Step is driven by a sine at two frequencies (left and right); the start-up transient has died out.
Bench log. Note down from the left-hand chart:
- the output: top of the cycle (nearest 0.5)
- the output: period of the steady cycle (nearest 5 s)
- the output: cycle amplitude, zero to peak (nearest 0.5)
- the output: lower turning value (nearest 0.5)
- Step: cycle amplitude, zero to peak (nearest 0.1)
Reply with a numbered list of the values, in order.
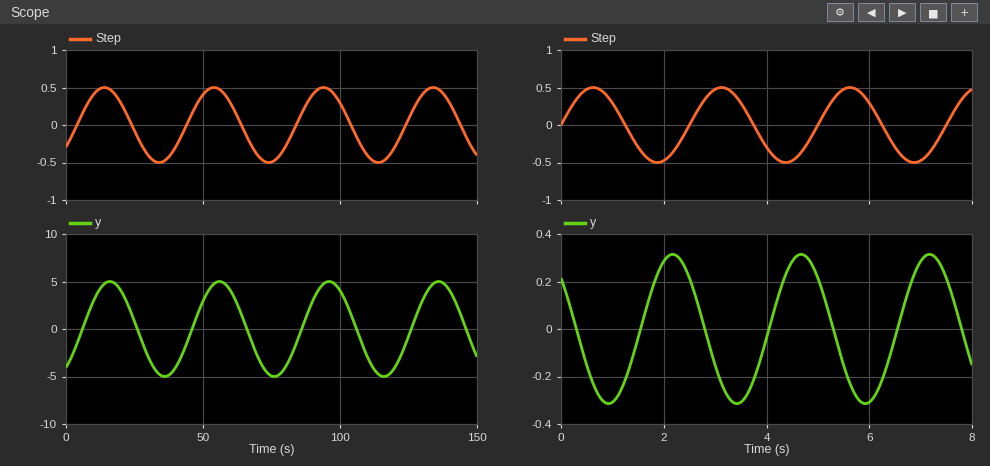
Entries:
1. 5.0
2. 40 s
3. 5.0
4. -5.0
5. 0.5
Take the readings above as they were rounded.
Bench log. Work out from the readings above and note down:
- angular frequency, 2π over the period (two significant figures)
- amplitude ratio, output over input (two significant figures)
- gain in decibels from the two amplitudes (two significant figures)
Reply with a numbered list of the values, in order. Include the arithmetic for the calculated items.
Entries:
1. 2π / 40 = 0.16 rad/s
2. 5 / 0.5 = 10
3. 20 log10(5 / 0.5) = 20 dB
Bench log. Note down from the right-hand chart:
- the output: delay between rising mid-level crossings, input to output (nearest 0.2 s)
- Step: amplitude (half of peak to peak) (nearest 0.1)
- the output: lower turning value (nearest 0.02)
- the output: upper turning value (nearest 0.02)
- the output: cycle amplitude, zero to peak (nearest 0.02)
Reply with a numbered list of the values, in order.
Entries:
1. 1.6 s
2. 0.5
3. -0.32
4. 0.32
5. 0.32
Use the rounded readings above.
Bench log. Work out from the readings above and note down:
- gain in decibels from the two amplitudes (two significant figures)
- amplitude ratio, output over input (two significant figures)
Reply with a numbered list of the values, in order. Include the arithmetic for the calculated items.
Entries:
1. 20 log10(0.32 / 0.5) = -3.9 dB
2. 0.32 / 0.5 = 0.64
